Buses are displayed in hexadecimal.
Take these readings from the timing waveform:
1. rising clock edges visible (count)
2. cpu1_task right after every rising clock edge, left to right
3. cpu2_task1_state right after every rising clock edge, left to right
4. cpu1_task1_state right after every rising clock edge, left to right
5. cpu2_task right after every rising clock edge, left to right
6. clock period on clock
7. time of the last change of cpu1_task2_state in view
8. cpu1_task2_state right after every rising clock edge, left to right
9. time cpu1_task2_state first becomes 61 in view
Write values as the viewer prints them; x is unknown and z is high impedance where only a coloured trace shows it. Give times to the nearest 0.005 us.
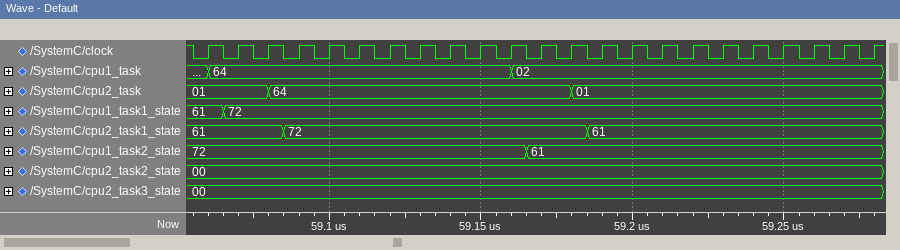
23
64, 64, 64, 64, 64, 64, 64, 64, 64, 64, 02, 02, 02, 02, 02, 02, 02, 02, 02, 02, 02, 02, 02
61, 61, 61, 72, 72, 72, 72, 72, 72, 72, 72, 72, 72, 61, 61, 61, 61, 61, 61, 61, 61, 61, 61
61, 72, 72, 72, 72, 72, 72, 72, 72, 72, 72, 72, 72, 72, 72, 72, 72, 72, 72, 72, 72, 72, 72
01, 01, 64, 64, 64, 64, 64, 64, 64, 64, 64, 64, 01, 01, 01, 01, 01, 01, 01, 01, 01, 01, 01
0.01 us
59.165 us
72, 72, 72, 72, 72, 72, 72, 72, 72, 72, 72, 61, 61, 61, 61, 61, 61, 61, 61, 61, 61, 61, 61
59.165 us
